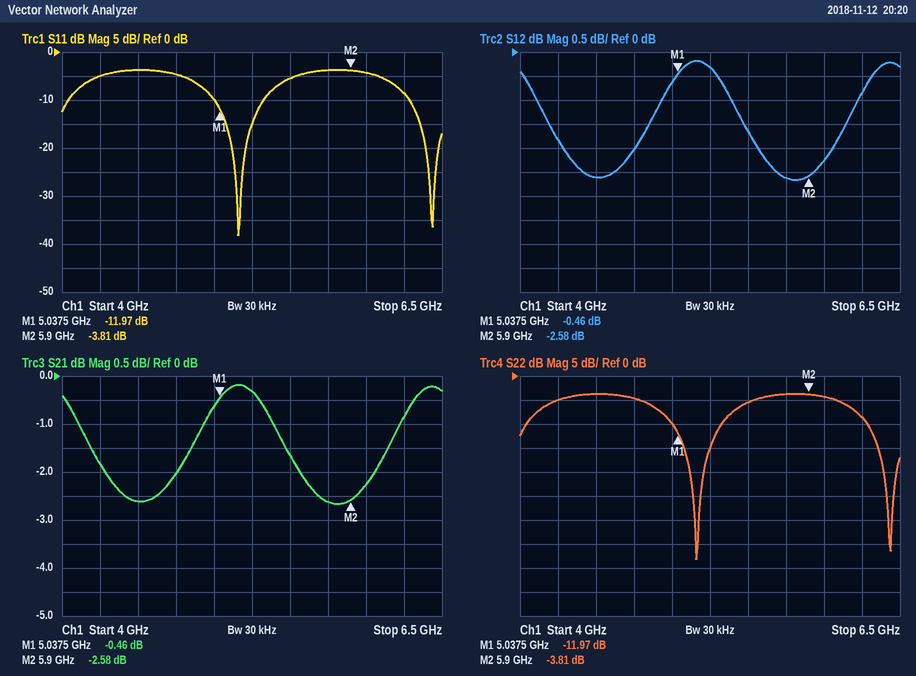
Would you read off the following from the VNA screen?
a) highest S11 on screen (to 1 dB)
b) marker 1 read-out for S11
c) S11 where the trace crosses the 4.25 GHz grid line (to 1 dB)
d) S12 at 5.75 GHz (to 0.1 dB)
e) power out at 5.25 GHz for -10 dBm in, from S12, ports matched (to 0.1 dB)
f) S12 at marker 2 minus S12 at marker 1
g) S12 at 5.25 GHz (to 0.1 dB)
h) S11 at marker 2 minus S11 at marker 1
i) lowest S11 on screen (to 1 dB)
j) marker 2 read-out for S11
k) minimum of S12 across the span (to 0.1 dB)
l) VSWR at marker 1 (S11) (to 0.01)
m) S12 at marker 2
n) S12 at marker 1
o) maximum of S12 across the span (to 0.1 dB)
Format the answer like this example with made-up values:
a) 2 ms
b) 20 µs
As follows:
a) -4 dB
b) -11.97 dB
c) -5 dB
d) -2.6 dB
e) -10.3 dBm
f) -2.12 dB
g) -0.3 dB
h) 8.16 dB
i) -38 dB
j) -3.81 dB
k) -2.7 dB
l) 1.67
m) -2.58 dB
n) -0.46 dB
o) -0.2 dB
